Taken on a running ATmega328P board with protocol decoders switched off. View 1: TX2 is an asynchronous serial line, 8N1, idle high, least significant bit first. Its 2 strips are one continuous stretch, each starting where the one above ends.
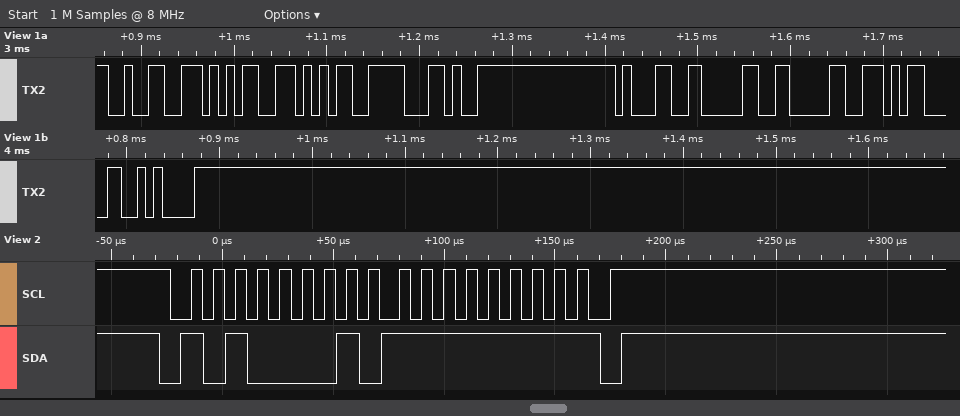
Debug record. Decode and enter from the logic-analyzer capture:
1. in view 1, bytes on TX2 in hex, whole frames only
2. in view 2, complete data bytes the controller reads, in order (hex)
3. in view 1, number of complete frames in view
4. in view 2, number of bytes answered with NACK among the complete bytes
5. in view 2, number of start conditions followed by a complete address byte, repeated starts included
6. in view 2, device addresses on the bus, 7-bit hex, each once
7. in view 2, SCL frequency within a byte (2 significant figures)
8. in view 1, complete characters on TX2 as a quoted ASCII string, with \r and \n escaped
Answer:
32 35 35 2C 31 30 30 0D 0A
FF
9
1
1
0x50
100 kHz
"255,100\r\n"
